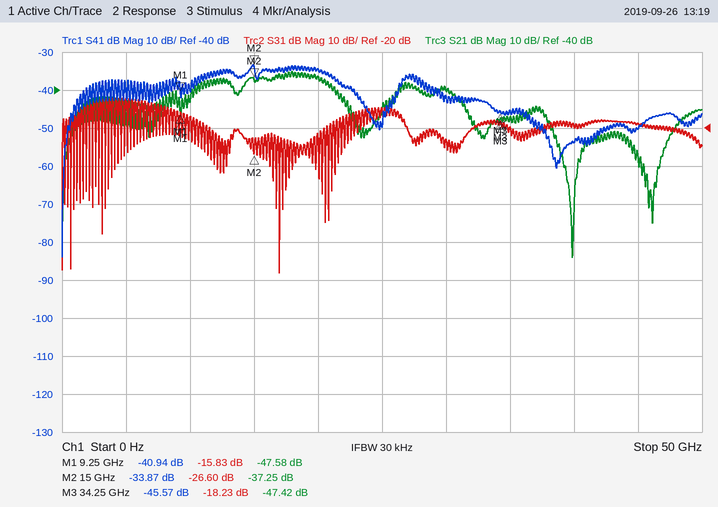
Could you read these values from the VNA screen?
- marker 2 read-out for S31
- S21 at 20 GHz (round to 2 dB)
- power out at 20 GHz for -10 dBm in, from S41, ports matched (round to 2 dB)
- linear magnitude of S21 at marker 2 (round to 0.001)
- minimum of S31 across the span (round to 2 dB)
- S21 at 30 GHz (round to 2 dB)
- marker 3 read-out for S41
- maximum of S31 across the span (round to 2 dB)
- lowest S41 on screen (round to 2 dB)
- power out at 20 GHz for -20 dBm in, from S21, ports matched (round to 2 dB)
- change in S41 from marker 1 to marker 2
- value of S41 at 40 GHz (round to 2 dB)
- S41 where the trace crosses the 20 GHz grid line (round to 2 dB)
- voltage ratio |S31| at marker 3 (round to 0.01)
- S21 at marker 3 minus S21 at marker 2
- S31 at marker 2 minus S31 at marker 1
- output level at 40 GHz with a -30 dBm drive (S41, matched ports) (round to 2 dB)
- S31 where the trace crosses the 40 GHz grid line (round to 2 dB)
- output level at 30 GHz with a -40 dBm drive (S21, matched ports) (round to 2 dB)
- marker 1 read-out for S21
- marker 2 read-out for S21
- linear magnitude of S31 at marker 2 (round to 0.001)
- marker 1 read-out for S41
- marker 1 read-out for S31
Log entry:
-26.60 dB
-36 dB
-44 dBm
0.014
-58 dB
-40 dB
-45.57 dB
-12 dB
-84 dB
-56 dBm
7.07 dB
-54 dB
-34 dB
0.12
-10.17 dB
-10.77 dB
-84 dBm
-20 dB
-80 dBm
-47.58 dB
-37.25 dB
0.047
-40.94 dB
-15.83 dB
